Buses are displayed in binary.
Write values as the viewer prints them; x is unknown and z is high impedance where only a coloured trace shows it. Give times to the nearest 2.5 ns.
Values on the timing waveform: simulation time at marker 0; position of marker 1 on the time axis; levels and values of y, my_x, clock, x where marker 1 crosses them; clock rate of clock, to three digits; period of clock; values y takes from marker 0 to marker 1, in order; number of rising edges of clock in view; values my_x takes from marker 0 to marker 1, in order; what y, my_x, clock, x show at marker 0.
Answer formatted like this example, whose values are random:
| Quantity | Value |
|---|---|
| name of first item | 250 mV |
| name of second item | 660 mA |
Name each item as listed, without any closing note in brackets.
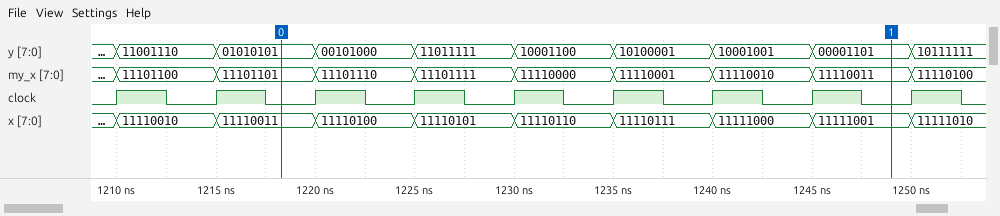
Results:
| Quantity | Value |
|---|---|
| simulation time at marker 0 | 1217.5 ns |
| position of marker 1 on the time axis | 1250 ns |
| levels and values of y, my_x, clock, x where marker 1 crosses them | y=00001101, my_x=11110011, clock=0, x=11111001 |
| clock rate of clock, to three digits | 200 MHz |
| period of clock | 5 ns |
| values y takes from marker 0 to marker 1, in order | 01010101, 00101000, 11011111, 10001100, 10100001, 10001001, 00001101 |
| number of rising edges of clock in view | 9 |
| values my_x takes from marker 0 to marker 1, in order | 11101101, 11101110, 11101111, 11110000, 11110001, 11110010, 11110011 |
| what y, my_x, clock, x show at marker 0 | y=01010101, my_x=11101101, clock=0, x=11110011 |
